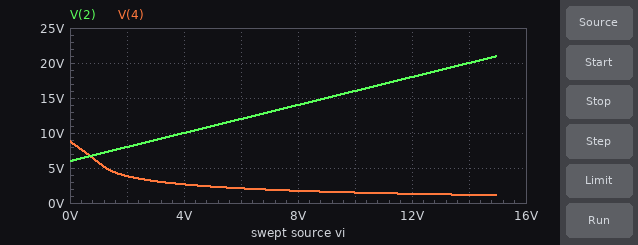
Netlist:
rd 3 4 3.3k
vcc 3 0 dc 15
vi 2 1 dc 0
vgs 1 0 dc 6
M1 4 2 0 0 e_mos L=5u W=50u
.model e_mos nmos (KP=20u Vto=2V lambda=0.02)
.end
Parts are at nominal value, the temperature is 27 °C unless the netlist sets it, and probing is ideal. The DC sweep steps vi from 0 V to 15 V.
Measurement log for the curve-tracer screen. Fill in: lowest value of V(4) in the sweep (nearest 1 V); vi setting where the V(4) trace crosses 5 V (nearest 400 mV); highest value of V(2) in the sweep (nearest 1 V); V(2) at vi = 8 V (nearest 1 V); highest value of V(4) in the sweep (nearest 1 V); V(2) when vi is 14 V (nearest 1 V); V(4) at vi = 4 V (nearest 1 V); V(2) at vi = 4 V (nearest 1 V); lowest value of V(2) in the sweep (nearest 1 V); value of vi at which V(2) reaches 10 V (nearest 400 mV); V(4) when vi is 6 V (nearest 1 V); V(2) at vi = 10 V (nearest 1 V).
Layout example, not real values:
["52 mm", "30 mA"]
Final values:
["1 V", "1.2 V", "21 V", "14 V", "9 V", "20 V", "3 V", "10 V", "6 V", "4.0 V", "2 V", "16 V"]
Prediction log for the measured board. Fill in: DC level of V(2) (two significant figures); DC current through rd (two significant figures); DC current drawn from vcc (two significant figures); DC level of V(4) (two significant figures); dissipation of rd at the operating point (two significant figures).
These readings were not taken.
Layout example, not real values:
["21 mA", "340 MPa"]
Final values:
["6.0 V", "1.9 mA", "1.9 mA", "8.8 V", "12 mW"]
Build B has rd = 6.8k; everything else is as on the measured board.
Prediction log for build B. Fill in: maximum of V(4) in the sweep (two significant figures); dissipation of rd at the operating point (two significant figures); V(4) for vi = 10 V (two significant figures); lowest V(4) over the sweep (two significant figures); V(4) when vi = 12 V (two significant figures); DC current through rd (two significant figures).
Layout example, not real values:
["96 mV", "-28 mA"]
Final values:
["3.5 V", "19 mW", "760 mV", "560 mV", "660 mV", "1.7 mA"]
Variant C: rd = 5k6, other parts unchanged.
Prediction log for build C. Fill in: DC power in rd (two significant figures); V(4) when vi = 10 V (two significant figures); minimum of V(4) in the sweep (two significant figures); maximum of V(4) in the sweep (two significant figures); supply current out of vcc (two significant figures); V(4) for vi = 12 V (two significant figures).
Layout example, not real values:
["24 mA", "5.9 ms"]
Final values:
["17 mW", "910 mV", "680 mV", "5.1 V", "1.8 mA", "800 mV"]
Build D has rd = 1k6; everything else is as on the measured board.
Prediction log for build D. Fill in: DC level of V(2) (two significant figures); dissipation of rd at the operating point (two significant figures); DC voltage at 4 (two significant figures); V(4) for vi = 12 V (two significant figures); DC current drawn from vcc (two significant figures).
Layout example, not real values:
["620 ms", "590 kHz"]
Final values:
["6.0 V", "6.3 mW", "12 V", "2.5 V", "2.0 mA"]
